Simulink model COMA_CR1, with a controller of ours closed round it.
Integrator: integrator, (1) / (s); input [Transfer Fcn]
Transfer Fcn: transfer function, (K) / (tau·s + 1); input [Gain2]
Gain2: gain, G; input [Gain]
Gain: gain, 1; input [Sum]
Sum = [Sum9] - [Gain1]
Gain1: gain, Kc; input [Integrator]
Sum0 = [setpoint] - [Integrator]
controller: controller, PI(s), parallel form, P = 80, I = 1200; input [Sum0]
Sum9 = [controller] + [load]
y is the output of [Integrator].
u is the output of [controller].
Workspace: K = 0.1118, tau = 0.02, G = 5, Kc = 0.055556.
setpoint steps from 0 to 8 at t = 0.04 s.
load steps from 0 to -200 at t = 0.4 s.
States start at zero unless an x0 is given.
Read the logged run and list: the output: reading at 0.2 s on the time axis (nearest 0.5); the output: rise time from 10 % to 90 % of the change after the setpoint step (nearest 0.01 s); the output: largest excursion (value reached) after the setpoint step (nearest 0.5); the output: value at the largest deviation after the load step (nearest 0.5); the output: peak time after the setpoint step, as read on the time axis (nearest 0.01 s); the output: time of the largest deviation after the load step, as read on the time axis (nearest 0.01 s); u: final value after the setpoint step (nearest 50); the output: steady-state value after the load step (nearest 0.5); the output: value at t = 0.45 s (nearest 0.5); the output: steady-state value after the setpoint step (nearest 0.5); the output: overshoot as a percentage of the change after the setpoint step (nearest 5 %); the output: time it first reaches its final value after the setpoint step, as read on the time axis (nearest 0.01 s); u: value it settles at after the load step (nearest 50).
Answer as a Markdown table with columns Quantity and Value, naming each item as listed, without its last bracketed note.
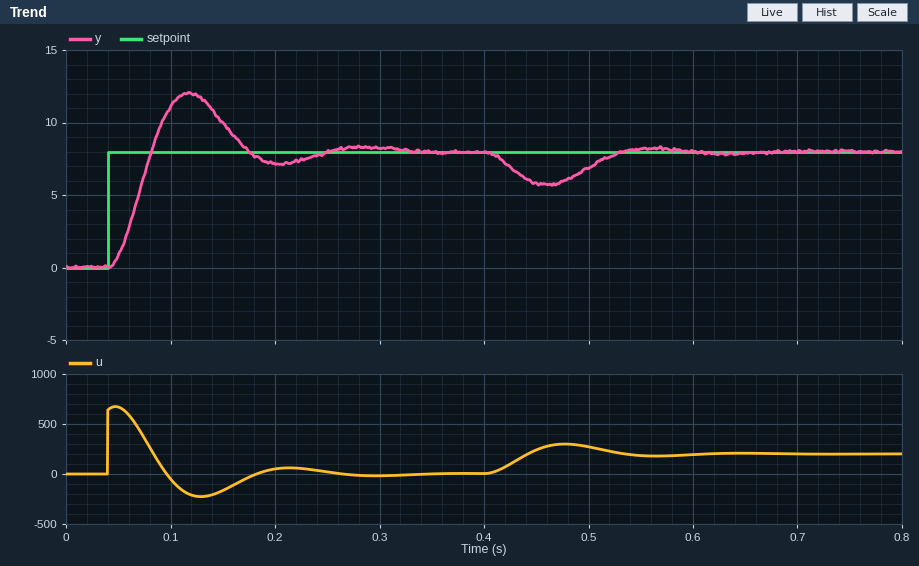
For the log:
| Quantity | Value |
|---|---|
| the output: reading at 0.2 s on the time axis | 7.0 |
| the output: rise time from 10 % to 90 % of the change after the setpoint step | 0.03 s |
| the output: largest excursion (value reached) after the setpoint step | 12.0 |
| the output: value at the largest deviation after the load step | 5.5 |
| the output: peak time after the setpoint step, as read on the time axis | 0.12 s |
| the output: time of the largest deviation after the load step, as read on the time axis | 0.46 s |
| u: final value after the setpoint step | 0 |
| the output: steady-state value after the load step | 8.0 |
| the output: value at t = 0.45 s | 6.0 |
| the output: steady-state value after the setpoint step | 8.0 |
| the output: overshoot as a percentage of the change after the setpoint step | 50 % |
| the output: time it first reaches its final value after the setpoint step, as read on the time axis | 0.08 s |
| u: value it settles at after the load step | 200 |
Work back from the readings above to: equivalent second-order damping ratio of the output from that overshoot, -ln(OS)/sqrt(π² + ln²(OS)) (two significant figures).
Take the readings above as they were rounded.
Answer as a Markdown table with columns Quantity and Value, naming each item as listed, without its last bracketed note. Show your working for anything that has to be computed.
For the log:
| Quantity | Value |
|---|---|
| equivalent second-order damping ratio of the output from that overshoot, -ln(OS)/sqrt(π² + ln²(OS)) | ln(0.5) = -0.693; 0.693 / sqrt(9.870 + 0.480) = 0.22 |
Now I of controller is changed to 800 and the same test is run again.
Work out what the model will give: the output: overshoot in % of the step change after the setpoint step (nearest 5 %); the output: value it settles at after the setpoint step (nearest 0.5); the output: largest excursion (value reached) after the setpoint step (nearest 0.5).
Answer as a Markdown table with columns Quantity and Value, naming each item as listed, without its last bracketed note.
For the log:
| Quantity | Value |
|---|---|
| the output: overshoot in % of the step change after the setpoint step | 40 % |
| the output: value it settles at after the setpoint step | 8.0 |
| the output: largest excursion (value reached) after the setpoint step | 11.0 |
